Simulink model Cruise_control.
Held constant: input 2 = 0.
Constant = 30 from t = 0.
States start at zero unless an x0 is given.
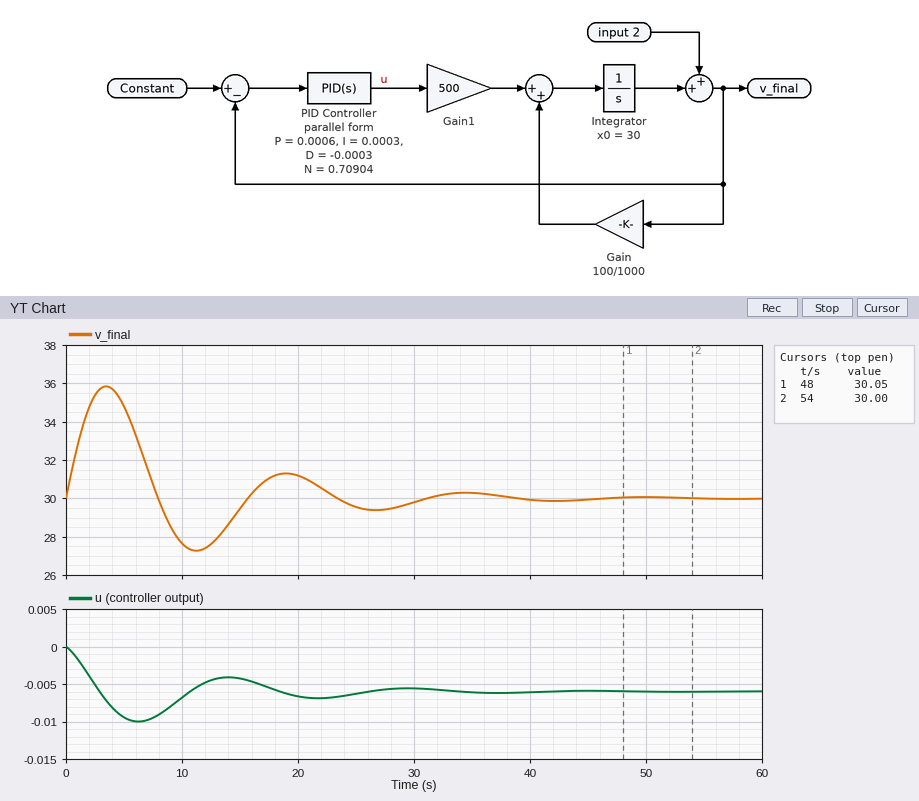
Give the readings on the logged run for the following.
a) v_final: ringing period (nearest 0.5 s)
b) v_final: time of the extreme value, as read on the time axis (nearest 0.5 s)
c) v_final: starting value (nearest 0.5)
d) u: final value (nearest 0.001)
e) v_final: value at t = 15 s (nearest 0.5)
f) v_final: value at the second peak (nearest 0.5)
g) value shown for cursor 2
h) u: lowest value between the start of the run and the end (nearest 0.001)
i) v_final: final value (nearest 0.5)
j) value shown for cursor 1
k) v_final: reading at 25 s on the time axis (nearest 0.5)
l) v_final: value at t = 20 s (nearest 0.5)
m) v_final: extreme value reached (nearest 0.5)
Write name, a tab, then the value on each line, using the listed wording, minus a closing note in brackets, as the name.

v_final: ringing period	15.5 s
v_final: time of the extreme value, as read on the time axis	3.5 s
v_final: starting value	30.0
u: final value	-0.006
v_final: value at t = 15 s	29.5
v_final: value at the second peak	31.5
value shown for cursor 2	30.00
u: lowest value between the start of the run and the end	-0.010
v_final: final value	30.0
value shown for cursor 1	30.05
v_final: reading at 25 s on the time axis	29.5
v_final: value at t = 20 s	31.0
v_final: extreme value reached	36.0
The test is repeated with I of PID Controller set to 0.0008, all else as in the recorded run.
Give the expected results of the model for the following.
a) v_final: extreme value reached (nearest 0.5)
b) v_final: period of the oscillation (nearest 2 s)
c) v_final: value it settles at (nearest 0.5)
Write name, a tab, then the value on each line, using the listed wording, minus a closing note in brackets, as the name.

v_final: extreme value reached	34.0
v_final: period of the oscillation	10 s
v_final: value it settles at	30.0
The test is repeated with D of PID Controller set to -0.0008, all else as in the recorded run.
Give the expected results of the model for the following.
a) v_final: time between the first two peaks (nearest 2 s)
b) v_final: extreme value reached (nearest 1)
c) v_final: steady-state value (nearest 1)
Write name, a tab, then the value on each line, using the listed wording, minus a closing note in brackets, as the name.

v_final: time between the first two peaks	14 s
v_final: extreme value reached	37
v_final: steady-state value	30
